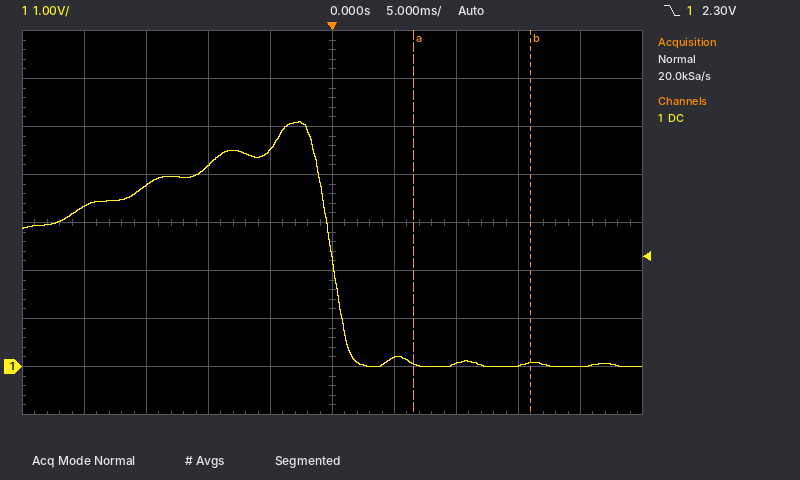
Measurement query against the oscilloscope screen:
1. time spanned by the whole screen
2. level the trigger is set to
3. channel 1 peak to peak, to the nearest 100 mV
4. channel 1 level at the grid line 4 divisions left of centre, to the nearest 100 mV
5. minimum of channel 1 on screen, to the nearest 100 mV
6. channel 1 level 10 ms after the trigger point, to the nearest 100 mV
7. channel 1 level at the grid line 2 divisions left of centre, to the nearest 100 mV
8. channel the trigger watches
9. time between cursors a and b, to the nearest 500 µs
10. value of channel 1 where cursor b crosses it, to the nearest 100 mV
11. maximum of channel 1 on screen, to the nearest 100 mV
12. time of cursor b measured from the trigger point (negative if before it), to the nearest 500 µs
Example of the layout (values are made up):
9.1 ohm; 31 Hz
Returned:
50 ms; 2.30 V; 5.1 V; 3.3 V; 0.0 V; 100 mV; 4.2 V; channel 1; 9.5 ms; 100 mV; 5.1 V; +16.0 ms
